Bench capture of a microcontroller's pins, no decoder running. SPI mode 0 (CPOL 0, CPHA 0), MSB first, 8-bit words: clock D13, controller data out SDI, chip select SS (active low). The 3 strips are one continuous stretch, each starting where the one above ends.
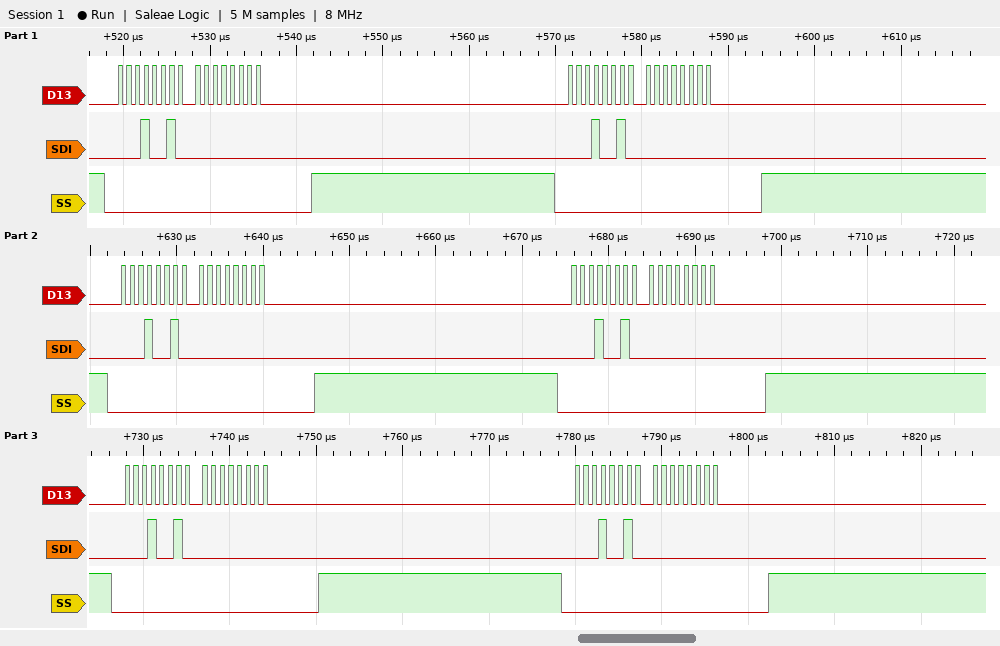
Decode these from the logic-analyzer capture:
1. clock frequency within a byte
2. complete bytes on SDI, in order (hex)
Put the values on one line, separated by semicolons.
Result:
1 MHz; 0x12 0x00 0x12 0x00 0x12 0x00 0x12 0x00 0x12 0x00 0x12 0x00
